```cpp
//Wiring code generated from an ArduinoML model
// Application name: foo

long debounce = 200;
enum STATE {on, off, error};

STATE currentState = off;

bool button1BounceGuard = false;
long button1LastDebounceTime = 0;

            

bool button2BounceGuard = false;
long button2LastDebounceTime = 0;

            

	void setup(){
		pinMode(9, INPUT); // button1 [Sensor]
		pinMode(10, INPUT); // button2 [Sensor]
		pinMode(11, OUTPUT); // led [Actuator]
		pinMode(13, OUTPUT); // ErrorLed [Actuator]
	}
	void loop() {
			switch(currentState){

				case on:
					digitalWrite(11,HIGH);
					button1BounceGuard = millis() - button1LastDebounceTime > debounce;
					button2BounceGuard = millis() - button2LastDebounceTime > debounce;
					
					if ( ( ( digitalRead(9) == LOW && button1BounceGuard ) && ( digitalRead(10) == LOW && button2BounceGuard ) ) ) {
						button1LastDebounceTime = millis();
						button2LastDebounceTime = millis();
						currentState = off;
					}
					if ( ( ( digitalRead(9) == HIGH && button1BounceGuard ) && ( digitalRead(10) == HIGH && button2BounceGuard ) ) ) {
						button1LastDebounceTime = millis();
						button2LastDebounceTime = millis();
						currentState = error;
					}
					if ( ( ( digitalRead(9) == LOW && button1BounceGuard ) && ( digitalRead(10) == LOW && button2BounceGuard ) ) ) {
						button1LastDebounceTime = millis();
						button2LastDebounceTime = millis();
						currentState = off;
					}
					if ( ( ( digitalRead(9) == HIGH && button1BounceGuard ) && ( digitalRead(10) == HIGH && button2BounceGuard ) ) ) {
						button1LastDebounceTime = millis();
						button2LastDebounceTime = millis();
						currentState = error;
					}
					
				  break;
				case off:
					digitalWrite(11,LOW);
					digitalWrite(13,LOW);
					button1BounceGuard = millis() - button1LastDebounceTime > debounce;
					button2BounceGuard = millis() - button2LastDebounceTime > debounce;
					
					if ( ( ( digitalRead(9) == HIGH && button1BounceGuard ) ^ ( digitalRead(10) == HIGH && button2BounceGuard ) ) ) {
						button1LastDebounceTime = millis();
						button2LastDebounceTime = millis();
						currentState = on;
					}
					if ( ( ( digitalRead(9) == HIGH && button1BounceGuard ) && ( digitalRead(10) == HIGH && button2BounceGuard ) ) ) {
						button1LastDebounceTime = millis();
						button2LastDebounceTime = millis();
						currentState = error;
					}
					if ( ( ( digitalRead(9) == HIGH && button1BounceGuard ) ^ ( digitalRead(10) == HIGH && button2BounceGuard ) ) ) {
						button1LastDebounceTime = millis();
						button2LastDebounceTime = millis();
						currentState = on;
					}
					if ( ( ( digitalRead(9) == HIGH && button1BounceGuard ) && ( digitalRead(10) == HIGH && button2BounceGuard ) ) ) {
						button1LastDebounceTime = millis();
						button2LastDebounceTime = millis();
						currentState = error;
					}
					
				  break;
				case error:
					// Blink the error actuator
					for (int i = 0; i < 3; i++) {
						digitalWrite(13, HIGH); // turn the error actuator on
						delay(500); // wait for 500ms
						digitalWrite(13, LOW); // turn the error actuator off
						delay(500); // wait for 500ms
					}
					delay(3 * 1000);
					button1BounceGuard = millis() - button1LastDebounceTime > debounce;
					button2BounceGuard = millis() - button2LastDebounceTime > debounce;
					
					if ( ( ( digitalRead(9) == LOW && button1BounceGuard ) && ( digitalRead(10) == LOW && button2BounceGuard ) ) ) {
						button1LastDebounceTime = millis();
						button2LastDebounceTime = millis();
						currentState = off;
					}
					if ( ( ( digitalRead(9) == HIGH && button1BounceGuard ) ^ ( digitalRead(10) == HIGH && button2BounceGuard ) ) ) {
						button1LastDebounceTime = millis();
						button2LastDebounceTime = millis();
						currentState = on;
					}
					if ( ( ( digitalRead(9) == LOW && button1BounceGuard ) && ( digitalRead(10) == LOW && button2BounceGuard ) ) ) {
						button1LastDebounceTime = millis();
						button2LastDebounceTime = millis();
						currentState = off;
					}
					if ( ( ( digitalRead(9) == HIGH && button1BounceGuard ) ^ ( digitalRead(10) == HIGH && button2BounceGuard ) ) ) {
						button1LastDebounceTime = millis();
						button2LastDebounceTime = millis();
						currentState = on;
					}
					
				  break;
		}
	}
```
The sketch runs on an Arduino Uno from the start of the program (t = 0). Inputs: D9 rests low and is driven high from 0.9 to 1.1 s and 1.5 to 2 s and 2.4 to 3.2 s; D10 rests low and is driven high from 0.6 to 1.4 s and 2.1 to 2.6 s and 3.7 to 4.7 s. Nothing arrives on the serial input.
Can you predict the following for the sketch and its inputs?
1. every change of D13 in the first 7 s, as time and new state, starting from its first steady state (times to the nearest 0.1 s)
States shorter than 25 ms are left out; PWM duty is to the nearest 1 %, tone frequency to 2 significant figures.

0 s low; 0.9 s high; 1.4 s low; 1.9 s high; 2.4 s low; 2.9 s high; 3.4 s low
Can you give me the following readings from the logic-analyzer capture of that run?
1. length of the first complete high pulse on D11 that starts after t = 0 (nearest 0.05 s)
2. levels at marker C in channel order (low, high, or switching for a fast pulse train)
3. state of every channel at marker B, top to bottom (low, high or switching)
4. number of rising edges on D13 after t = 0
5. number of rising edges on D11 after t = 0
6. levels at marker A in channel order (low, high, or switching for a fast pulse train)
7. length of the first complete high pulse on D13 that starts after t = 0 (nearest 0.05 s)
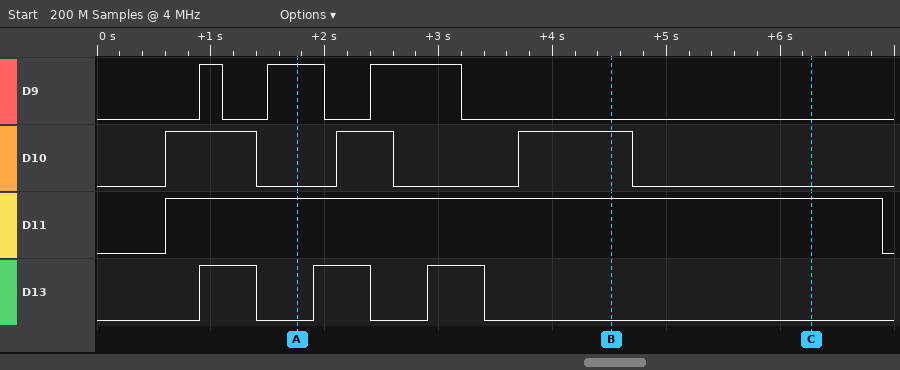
6.30 s
D9 low, D10 low, D11 high, D13 low
D9 low, D10 high, D11 high, D13 low
3
1
D9 high, D10 low, D11 high, D13 low
0.50 s
